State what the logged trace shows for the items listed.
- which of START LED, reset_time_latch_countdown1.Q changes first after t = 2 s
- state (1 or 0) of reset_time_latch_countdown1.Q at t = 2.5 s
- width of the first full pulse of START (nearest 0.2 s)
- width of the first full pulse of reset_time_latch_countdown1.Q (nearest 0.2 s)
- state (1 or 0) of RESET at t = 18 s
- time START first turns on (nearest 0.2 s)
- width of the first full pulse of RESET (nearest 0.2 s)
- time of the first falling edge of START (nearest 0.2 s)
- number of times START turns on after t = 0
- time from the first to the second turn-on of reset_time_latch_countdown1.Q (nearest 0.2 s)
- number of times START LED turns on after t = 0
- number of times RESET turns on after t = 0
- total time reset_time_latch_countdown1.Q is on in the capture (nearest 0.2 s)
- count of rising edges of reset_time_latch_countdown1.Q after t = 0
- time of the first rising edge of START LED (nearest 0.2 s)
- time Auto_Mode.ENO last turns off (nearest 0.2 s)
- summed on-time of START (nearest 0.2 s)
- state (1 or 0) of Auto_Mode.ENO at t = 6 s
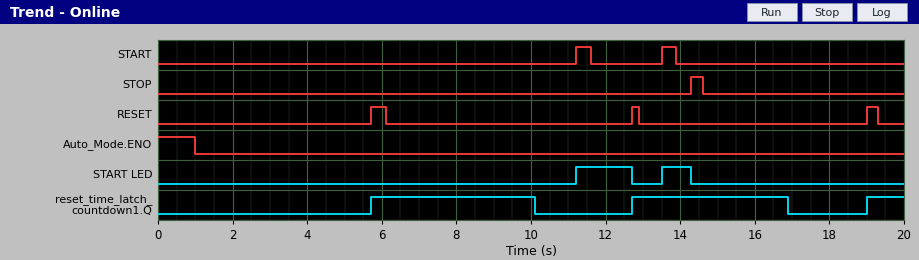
reset_time_latch_countdown1.Q
0
0.4 s
4.4 s
0
11.2 s
0.4 s
11.6 s
2
7.0 s
2
3
9.6 s
3
11.2 s
1.0 s
0.8 s
0
